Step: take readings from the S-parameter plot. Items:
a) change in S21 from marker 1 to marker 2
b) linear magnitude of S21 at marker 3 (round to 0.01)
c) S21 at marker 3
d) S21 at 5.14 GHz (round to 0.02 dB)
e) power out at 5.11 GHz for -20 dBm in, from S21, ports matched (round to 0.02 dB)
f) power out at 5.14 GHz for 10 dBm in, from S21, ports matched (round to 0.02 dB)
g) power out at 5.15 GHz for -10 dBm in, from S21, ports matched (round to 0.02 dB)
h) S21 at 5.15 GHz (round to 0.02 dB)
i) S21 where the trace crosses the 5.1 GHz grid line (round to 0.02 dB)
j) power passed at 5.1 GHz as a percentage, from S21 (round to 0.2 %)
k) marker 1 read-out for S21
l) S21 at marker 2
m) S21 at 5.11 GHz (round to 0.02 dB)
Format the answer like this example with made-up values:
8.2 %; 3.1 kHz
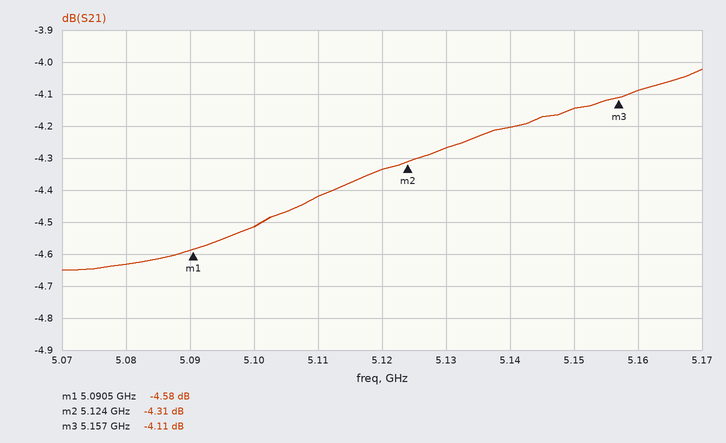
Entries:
0.27 dB; 0.62; -4.11 dB; -4.20 dB; -24.42 dBm; 5.80 dBm; -14.14 dBm; -4.14 dB; -4.52 dB; 35.4 %; -4.58 dB; -4.31 dB; -4.42 dB
